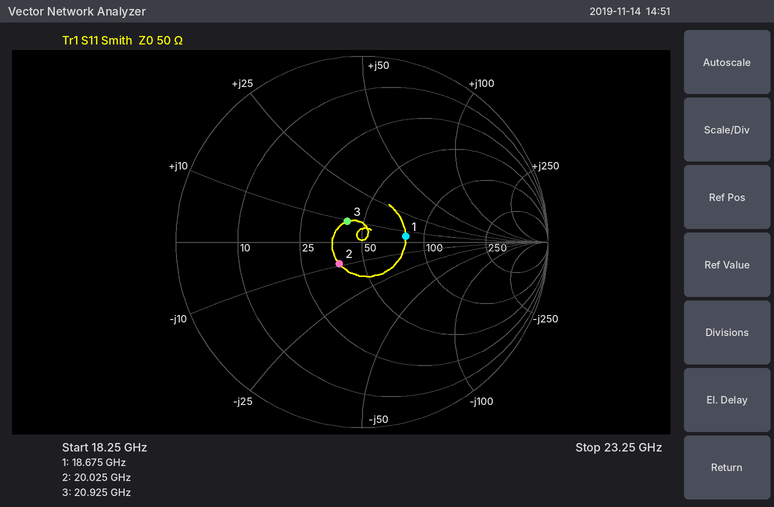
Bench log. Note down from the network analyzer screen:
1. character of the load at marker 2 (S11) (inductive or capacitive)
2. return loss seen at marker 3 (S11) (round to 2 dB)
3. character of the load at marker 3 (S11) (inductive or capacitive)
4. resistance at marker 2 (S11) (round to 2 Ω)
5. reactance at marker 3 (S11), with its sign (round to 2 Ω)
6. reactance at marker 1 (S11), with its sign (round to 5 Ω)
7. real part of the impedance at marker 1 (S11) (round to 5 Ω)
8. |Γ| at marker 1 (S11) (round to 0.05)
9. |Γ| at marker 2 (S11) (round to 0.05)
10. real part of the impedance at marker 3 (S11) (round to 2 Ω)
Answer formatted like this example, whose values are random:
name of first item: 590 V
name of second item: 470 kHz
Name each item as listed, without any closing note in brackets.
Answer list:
character of the load at marker 2 (S11): capacitive
return loss seen at marker 3 (S11): 18 dB
character of the load at marker 3 (S11): inductive
resistance at marker 2 (S11): 38 Ω
reactance at marker 3 (S11), with its sign: +10 Ω
reactance at marker 1 (S11), with its sign: +5 Ω
real part of the impedance at marker 1 (S11): 80 Ω
|Γ| at marker 1 (S11): 0.25
|Γ| at marker 2 (S11): 0.15
real part of the impedance at marker 3 (S11): 42 Ω
